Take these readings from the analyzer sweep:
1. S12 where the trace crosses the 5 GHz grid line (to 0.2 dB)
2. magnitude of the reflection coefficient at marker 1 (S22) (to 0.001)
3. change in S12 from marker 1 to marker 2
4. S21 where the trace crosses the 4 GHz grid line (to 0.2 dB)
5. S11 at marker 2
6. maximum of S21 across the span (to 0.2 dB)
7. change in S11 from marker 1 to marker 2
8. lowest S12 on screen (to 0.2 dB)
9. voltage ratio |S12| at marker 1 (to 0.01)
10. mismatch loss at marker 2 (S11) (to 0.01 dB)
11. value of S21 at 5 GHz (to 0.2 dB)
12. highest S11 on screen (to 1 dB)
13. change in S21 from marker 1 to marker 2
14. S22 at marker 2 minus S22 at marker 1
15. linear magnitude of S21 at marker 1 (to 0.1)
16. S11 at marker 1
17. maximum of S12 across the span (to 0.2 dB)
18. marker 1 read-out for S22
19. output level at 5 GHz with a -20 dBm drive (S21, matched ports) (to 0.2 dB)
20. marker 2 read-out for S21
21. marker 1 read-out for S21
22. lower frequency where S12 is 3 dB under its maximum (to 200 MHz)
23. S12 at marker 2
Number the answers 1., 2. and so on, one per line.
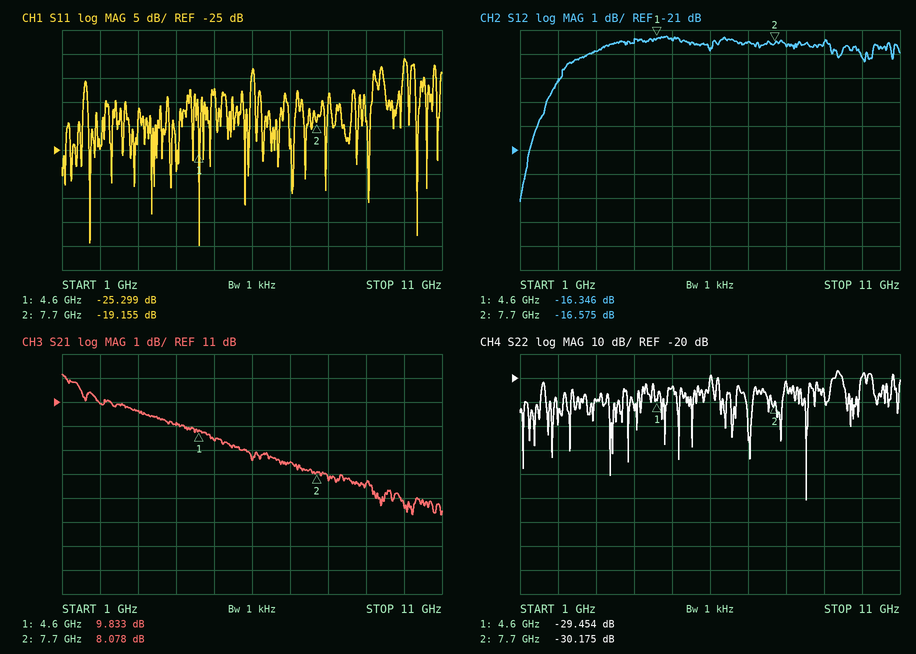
1. -16.4 dB
2. 0.034
3. -0.229 dB
4. 10.0 dB
5. -19.155 dB
6. 12.2 dB
7. 6.144 dB
8. -23.2 dB
9. 0.15
10. 0.05 dB
11. 9.4 dB
12. -6 dB
13. -1.755 dB
14. -0.721 dB
15. 3.1
16. -25.299 dB
17. -16.2 dB
18. -29.454 dB
19. -10.6 dBm
20. 8.078 dB
21. 9.833 dB
22. 1.6 GHz
23. -16.575 dB
